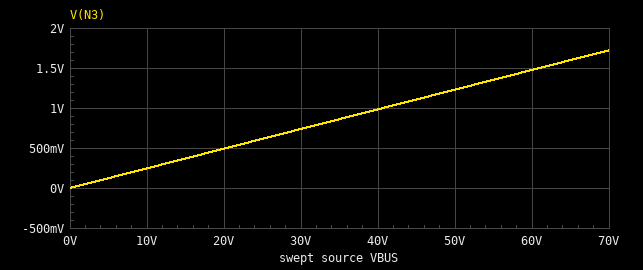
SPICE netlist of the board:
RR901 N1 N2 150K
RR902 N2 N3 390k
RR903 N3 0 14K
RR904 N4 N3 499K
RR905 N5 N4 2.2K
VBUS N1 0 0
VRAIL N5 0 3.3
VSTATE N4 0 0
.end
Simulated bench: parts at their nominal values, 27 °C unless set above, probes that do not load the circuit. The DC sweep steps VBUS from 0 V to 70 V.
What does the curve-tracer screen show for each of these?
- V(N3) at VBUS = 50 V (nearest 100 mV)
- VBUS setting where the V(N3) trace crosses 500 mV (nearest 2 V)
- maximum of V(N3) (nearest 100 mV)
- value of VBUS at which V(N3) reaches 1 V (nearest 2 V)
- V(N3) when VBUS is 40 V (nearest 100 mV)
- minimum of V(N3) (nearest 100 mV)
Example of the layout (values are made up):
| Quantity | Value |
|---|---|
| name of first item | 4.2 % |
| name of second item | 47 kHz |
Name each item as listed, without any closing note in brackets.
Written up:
| Quantity | Value |
|---|---|
| V(N3) at VBUS = 50 V | 1.2 V |
| VBUS setting where the V(N3) trace crosses 500 mV | 20 V |
| maximum of V(N3) | 1.7 V |
| value of VBUS at which V(N3) reaches 1 V | 40 V |
| V(N3) when VBUS is 40 V | 1.0 V |
| minimum of V(N3) | 0 V |
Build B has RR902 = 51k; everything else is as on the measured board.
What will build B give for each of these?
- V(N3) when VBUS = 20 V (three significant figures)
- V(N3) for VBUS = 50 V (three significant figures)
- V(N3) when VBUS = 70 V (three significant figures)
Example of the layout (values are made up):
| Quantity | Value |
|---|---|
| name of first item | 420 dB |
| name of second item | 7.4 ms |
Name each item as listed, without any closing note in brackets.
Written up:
| Quantity | Value |
|---|---|
| V(N3) when VBUS = 20 V | 1.27 V |
| V(N3) for VBUS = 50 V | 3.17 V |
| V(N3) when VBUS = 70 V | 4.44 V |
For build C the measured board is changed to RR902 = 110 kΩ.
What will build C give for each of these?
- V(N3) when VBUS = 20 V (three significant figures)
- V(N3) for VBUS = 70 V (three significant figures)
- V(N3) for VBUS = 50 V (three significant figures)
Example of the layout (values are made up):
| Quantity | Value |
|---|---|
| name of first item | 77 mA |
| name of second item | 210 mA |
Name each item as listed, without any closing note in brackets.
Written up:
| Quantity | Value |
|---|---|
| V(N3) when VBUS = 20 V | 995 mV |
| V(N3) for VBUS = 70 V | 3.48 V |
| V(N3) for VBUS = 50 V | 2.49 V |
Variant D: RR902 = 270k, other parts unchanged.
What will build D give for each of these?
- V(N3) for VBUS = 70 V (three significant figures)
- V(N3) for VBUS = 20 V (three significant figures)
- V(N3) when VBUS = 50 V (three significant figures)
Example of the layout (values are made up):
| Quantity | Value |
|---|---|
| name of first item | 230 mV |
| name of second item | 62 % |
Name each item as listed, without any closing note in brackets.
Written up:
| Quantity | Value |
|---|---|
| V(N3) for VBUS = 70 V | 2.20 V |
| V(N3) for VBUS = 20 V | 628 mV |
| V(N3) when VBUS = 50 V | 1.57 V |
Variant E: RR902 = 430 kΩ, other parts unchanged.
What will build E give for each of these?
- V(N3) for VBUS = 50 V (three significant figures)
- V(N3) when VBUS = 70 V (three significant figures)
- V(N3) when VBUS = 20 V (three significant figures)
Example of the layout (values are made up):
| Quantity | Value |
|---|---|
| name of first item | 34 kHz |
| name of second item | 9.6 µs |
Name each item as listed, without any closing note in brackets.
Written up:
| Quantity | Value |
|---|---|
| V(N3) for VBUS = 50 V | 1.15 V |
| V(N3) when VBUS = 70 V | 1.61 V |
| V(N3) when VBUS = 20 V | 459 mV |
